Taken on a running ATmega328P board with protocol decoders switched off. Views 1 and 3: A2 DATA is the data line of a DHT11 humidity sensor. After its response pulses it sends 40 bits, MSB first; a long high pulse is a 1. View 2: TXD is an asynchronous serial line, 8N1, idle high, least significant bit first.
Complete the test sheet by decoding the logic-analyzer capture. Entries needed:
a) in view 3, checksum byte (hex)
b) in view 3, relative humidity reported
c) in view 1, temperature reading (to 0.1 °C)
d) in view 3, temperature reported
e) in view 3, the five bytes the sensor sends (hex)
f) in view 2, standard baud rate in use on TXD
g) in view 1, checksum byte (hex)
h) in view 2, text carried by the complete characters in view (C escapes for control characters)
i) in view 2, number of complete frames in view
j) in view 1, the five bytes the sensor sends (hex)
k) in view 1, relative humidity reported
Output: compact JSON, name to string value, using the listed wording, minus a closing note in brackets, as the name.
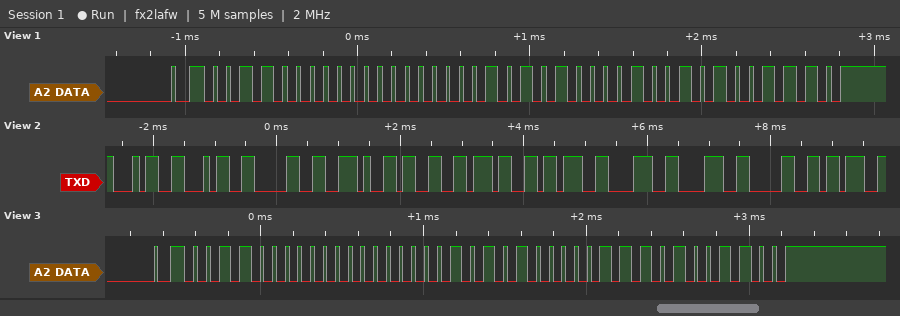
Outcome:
{"in view 3, checksum byte": "0x4C", "in view 3, relative humidity reported": "48 %", "in view 1, temperature reading": "21.9 °C", "in view 3, temperature reported": "21.7 °C", "in view 3, the five bytes the sensor sends": "30 00 15 07 4C", "in view 2, standard baud rate in use on TXD": "9600 baud", "in view 1, checksum byte": "0x4E", "in view 2, text carried by the complete characters in view": "\"440.37;880;\"", "in view 2, number of complete frames in view": "11", "in view 1, the five bytes the sensor sends": "30 00 15 09 4E", "in view 1, relative humidity reported": "48 %"}
